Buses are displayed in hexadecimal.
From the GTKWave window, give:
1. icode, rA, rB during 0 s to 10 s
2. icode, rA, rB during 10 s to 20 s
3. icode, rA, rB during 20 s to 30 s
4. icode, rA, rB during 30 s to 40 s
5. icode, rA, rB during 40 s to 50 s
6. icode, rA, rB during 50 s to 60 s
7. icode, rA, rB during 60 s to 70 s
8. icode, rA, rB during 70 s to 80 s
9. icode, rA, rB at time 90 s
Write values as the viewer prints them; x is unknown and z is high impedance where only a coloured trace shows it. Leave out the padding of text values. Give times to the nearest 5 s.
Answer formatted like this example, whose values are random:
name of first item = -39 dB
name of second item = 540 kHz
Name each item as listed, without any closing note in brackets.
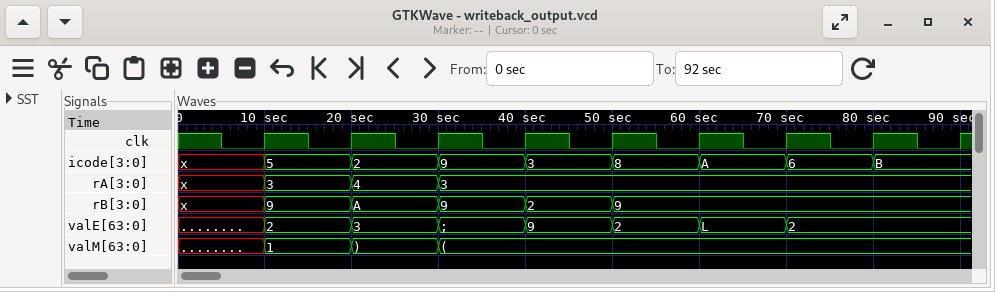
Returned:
icode, rA, rB during 0 s to 10 s = icode=x, rA=x, rB=x
icode, rA, rB during 10 s to 20 s = icode=5, rA=3, rB=9
icode, rA, rB during 20 s to 30 s = icode=2, rA=4, rB=A
icode, rA, rB during 30 s to 40 s = icode=9, rA=3, rB=9
icode, rA, rB during 40 s to 50 s = icode=3, rA=3, rB=2
icode, rA, rB during 50 s to 60 s = icode=8, rA=3, rB=9
icode, rA, rB during 60 s to 70 s = icode=A, rA=3, rB=9
icode, rA, rB during 70 s to 80 s = icode=6, rA=3, rB=9
icode, rA, rB at time 90 s = icode=B, rA=3, rB=9
